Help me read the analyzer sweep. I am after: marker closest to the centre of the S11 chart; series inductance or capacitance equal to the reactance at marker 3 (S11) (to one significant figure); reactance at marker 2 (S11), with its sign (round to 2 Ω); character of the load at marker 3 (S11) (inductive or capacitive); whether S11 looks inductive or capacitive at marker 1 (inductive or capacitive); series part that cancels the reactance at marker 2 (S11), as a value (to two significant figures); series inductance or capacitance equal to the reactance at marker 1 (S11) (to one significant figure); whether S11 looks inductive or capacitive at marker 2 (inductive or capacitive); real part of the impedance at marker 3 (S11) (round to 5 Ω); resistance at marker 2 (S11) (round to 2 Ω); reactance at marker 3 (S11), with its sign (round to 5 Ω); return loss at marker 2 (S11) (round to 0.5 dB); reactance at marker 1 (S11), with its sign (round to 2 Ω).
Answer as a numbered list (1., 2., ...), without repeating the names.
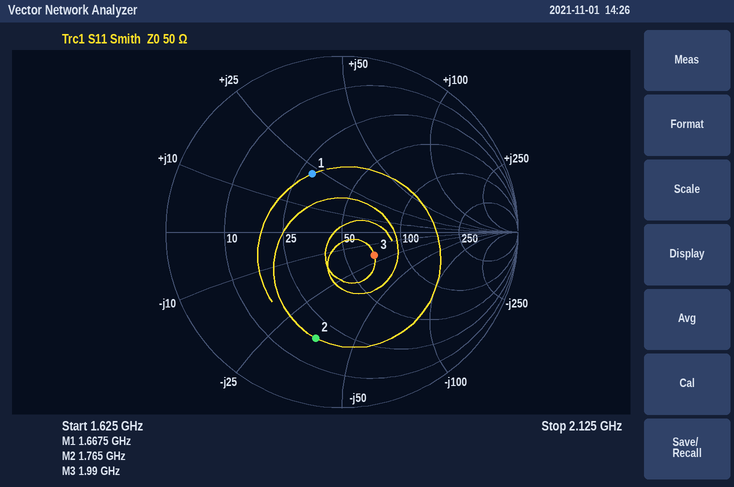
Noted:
1. marker 3
2. 4 pF
3. -36 Ω
4. capacitive
5. inductive
6. 3.2 nH
7. 2 nH
8. capacitive
9. 70 Ω
10. 18 Ω
11. -20 Ω
12. 4.0 dB
13. +22 Ω
